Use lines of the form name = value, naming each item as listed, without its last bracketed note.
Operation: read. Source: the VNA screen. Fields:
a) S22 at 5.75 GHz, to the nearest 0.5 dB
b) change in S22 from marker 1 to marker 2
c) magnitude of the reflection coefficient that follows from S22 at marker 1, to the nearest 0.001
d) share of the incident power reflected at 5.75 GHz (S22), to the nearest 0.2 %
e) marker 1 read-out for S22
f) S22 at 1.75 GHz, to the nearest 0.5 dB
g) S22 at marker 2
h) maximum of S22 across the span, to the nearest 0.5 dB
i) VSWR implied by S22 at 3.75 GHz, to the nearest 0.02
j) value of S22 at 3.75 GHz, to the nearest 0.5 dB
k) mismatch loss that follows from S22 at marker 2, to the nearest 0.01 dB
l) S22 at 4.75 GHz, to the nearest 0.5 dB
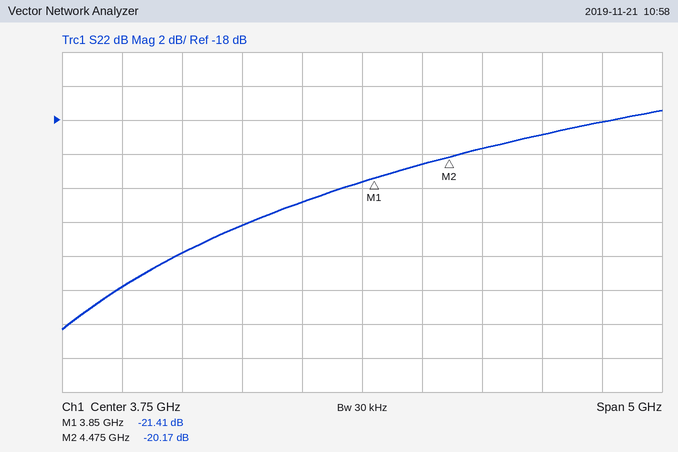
S22 at 5.75 GHz, to the nearest 0.5 dB = -18.0 dB
change in S22 from marker 1 to marker 2 = 1.24 dB
magnitude of the reflection coefficient that follows from S22 at marker 1, to the nearest 0.001 = 0.085
share of the incident power reflected at 5.75 GHz (S22), to the nearest 0.2 % = 1.6 %
marker 1 read-out for S22 = -21.41 dB
S22 at 1.75 GHz, to the nearest 0.5 dB = -28.0 dB
S22 at marker 2 = -20.17 dB
maximum of S22 across the span, to the nearest 0.5 dB = -17.5 dB
VSWR implied by S22 at 3.75 GHz, to the nearest 0.02 = 1.18
value of S22 at 3.75 GHz, to the nearest 0.5 dB = -21.5 dB
mismatch loss that follows from S22 at marker 2, to the nearest 0.01 dB = 0.04 dB
S22 at 4.75 GHz, to the nearest 0.5 dB = -19.5 dB
